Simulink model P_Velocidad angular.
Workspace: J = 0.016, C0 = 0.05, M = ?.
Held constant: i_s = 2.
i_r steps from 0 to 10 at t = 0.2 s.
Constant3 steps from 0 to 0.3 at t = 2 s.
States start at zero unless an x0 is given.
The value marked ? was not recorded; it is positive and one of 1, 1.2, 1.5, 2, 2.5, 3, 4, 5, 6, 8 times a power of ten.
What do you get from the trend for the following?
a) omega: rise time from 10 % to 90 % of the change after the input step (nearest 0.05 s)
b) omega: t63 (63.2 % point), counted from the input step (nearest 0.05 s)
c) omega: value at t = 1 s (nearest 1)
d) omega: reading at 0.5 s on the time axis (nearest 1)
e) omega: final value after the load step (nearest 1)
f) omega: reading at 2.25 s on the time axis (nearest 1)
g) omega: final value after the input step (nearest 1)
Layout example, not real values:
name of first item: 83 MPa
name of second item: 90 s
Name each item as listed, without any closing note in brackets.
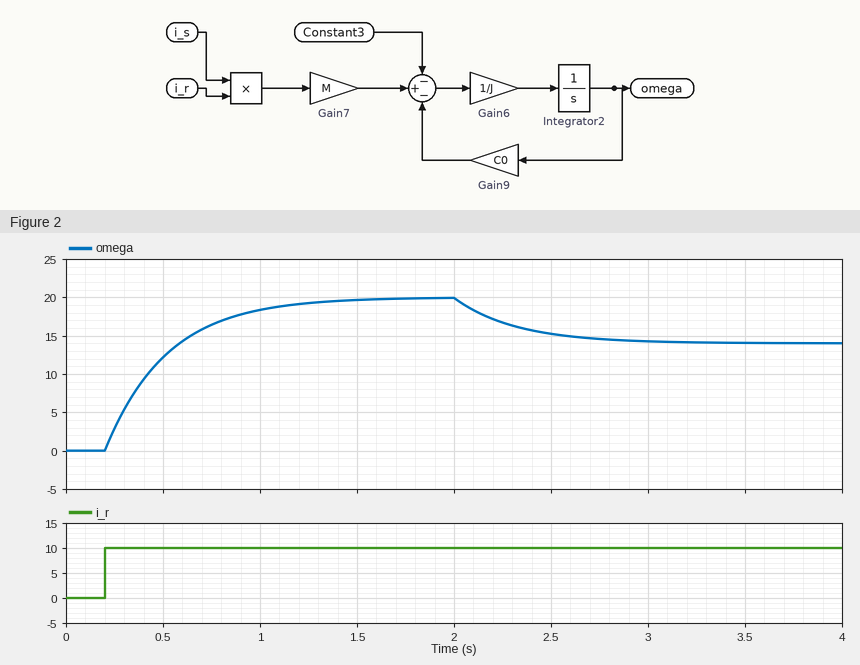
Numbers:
omega: rise time from 10 % to 90 % of the change after the input step: 0.70 s
omega: t63 (63.2 % point), counted from the input step: 0.30 s
omega: value at t = 1 s: 18
omega: reading at 0.5 s on the time axis: 12
omega: final value after the load step: 14
omega: reading at 2.25 s on the time axis: 17
omega: final value after the input step: 20
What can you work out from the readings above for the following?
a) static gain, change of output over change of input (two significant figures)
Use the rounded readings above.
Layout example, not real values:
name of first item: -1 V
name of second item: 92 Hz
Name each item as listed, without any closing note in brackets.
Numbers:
static gain, change of output over change of input: 2.0
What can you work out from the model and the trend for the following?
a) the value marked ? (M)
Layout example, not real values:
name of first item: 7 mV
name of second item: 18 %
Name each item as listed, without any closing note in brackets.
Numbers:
the value marked ?: 0.05
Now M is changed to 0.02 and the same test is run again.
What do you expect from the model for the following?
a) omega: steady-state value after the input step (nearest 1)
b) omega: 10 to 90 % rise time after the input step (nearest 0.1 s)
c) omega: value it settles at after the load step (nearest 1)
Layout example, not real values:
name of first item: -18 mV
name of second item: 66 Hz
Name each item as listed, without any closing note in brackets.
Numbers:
omega: steady-state value after the input step: 8
omega: 10 to 90 % rise time after the input step: 0.7 s
omega: value it settles at after the load step: 2
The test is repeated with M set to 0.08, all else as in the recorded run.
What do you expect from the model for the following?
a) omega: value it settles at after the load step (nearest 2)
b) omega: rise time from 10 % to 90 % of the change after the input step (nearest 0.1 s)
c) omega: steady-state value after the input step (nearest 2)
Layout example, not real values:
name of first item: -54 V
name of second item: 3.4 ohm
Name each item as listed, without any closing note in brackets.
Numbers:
omega: value it settles at after the load step: 26
omega: rise time from 10 % to 90 % of the change after the input step: 0.7 s
omega: steady-state value after the input step: 32
